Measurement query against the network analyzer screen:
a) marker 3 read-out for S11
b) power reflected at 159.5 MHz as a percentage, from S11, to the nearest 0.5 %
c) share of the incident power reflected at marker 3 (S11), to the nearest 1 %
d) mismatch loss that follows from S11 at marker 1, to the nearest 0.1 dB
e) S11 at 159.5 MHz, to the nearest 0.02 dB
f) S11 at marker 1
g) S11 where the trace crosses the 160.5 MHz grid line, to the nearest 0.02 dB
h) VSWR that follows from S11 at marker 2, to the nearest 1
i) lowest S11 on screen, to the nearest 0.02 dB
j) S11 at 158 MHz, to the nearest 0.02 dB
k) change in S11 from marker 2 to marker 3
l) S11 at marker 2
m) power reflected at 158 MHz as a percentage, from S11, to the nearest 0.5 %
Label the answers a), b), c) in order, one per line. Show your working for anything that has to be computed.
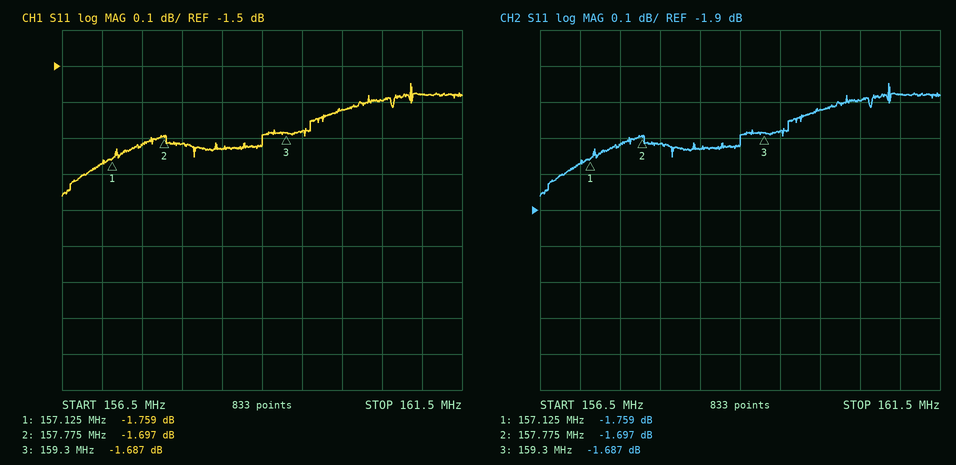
a) -1.687 dB
b) 10^(-1.68/10) ≈ 67.9 %, so 68.0 % to the nearest 0.5 %
c) 10^(-1.687/10) ≈ 68 %
d) −10 log10(1 − 10^(-1.759/10)) ≈ 4.8 dB
e) -1.68 dB
f) -1.759 dB
g) -1.60 dB
h) (1 + 0.8225)/(1 − 0.8225) ≈ 10
i) -1.86 dB
j) -1.72 dB
k) -1.687 − (-1.697) = 0.010 dB
l) -1.697 dB
m) 10^(-1.72/10) ≈ 67.3 %, so 67.5 % to the nearest 0.5 %
